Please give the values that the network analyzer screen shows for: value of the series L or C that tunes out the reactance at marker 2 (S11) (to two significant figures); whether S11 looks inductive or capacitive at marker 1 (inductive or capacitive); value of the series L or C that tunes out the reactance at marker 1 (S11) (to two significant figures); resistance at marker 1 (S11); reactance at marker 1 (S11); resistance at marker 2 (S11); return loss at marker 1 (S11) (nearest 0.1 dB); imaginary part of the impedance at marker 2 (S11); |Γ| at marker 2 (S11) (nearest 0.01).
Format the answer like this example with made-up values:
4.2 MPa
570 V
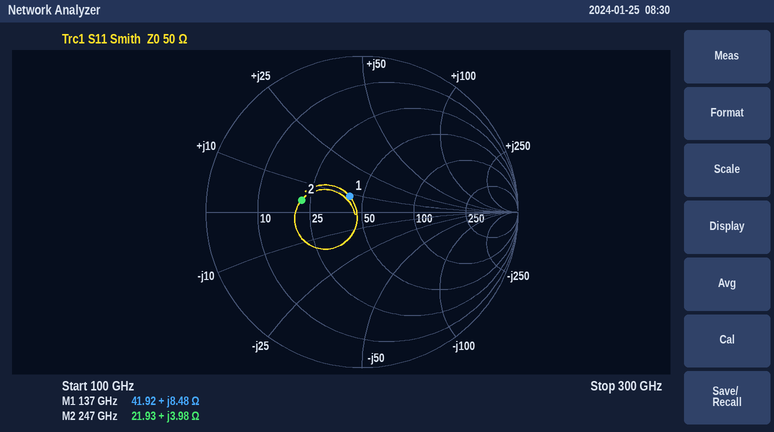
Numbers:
160 fF
inductive
140 fF
41.92 Ω
+8.48 Ω
21.93 Ω
17.9 dB
+3.98 Ω
0.39
